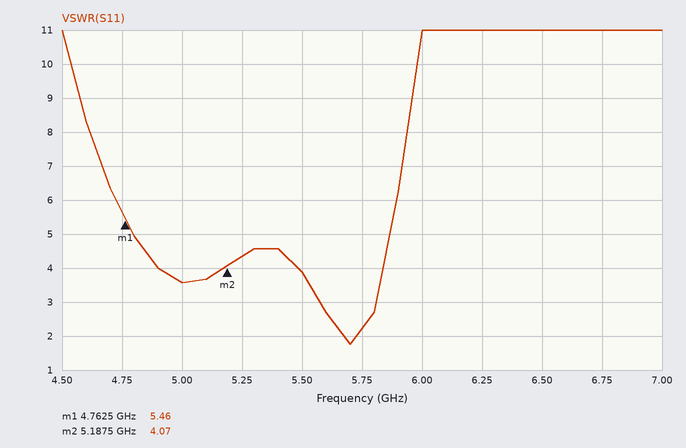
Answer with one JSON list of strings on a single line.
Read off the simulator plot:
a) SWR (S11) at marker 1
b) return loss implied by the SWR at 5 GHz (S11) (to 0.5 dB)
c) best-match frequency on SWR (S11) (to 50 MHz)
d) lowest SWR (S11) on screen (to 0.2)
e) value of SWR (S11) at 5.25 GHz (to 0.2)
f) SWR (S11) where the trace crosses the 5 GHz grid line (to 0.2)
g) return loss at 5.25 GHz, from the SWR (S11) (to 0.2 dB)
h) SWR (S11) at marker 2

["5.46", "5.0 dB", "5.70 GHz", "1.8", "4.4", "3.6", "4.0 dB", "4.07"]
